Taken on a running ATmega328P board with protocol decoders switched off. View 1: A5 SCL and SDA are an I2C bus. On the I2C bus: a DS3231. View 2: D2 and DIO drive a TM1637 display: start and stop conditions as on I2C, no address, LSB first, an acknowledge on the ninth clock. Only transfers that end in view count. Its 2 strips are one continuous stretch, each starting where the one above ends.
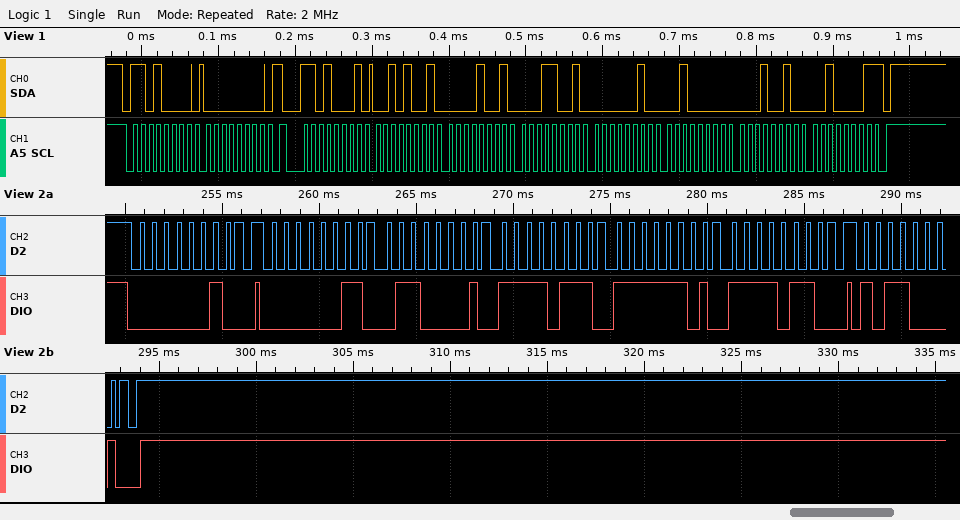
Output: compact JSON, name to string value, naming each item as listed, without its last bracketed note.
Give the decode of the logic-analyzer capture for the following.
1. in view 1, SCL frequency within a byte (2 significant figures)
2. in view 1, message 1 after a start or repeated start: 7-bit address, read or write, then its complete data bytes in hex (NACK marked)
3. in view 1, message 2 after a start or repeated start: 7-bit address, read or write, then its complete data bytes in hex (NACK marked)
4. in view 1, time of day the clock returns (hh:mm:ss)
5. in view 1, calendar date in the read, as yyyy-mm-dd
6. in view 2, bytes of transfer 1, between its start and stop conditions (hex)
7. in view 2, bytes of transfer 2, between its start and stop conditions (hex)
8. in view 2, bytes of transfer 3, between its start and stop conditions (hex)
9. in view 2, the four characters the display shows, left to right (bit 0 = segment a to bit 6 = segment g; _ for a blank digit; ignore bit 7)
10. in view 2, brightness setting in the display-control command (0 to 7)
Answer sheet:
{"in view 1, SCL frequency within a byte": "100 kHz", "in view 1, message 1 after a start or repeated start: 7-bit address, read or write, then its complete data bytes in hex": "0x68 write: 00", "in view 1, message 2 after a start or repeated start: 7-bit address, read or write, then its complete data bytes in hex": "0x68 read: 29 09 19 02 20 12 21 NACK", "in view 1, time of day the clock returns": "19:09:29", "in view 1, calendar date in the read, as yyyy-mm-dd": "2021-12-20", "in view 2, bytes of transfer 1, between its start and stop conditions": "40", "in view 2, bytes of transfer 2, between its start and stop conditions": "C0 86 EF BF 6F", "in view 2, bytes of transfer 3, between its start and stop conditions": "8D", "in view 2, the four characters the display shows, left to right": "1909", "in view 2, brightness setting in the display-control command": "5"}
